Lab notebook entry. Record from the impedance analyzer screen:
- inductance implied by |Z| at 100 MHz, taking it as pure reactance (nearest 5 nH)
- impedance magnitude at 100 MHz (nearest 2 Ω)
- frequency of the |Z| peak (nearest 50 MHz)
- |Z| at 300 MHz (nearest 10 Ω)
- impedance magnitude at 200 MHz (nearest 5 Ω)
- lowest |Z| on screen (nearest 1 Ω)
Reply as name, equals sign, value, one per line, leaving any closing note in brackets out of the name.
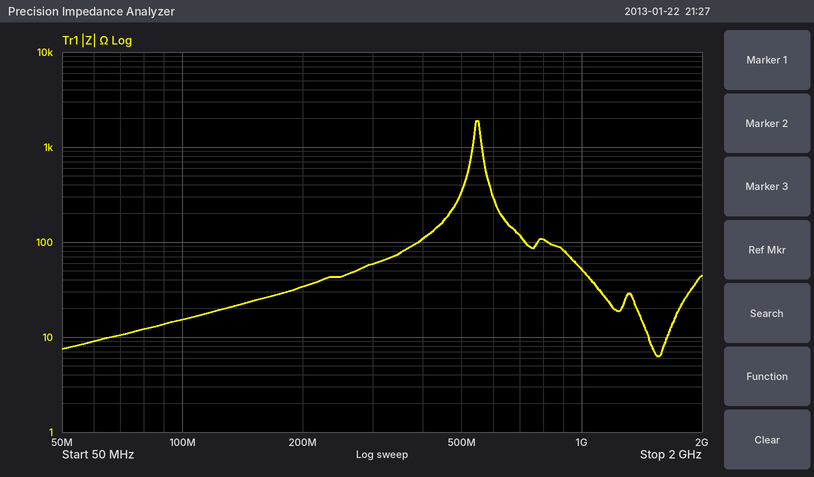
inductance implied by |Z| at 100 MHz, taking it as pure reactance = 25 nH
impedance magnitude at 100 MHz = 16 Ω
frequency of the |Z| peak = 550 MHz
|Z| at 300 MHz = 60 Ω
impedance magnitude at 200 MHz = 35 Ω
lowest |Z| on screen = 6 Ω
